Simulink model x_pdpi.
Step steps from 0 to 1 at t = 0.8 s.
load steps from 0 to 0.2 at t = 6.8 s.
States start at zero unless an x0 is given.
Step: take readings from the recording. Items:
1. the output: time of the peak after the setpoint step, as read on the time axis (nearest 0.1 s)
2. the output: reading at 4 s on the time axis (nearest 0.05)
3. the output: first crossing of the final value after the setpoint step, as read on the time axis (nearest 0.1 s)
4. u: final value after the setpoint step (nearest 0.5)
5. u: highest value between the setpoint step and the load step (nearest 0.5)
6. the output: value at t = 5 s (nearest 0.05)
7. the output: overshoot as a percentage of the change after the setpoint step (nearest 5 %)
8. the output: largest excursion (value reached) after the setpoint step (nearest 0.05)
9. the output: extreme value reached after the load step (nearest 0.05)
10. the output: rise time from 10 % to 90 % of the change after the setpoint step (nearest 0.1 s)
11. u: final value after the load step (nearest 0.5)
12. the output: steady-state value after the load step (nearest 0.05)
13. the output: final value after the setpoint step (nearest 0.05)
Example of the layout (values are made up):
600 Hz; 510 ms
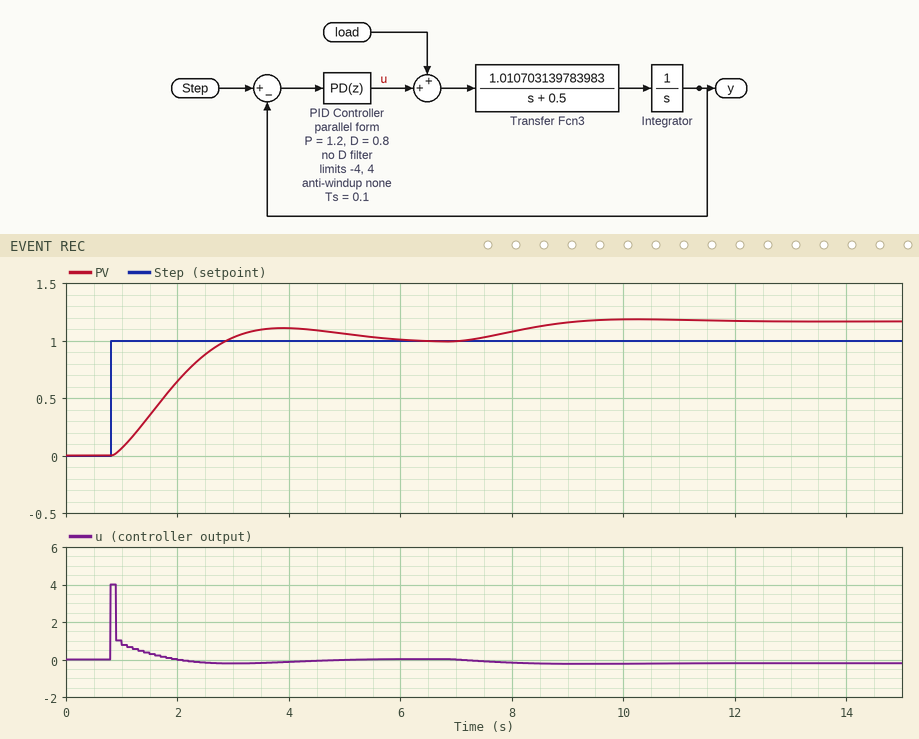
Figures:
3.9 s; 1.10; 2.9 s; 0.0; 4.0; 1.05; 10 %; 1.10; 1.20; 1.5 s; 0.0; 1.15; 1.00
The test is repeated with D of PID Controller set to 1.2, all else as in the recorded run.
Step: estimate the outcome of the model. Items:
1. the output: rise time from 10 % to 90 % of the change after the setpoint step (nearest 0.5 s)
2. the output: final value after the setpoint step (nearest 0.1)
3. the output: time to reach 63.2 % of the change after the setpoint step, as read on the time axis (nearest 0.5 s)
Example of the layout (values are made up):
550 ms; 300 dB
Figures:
2.0 s; 1.0; 2.0 s
